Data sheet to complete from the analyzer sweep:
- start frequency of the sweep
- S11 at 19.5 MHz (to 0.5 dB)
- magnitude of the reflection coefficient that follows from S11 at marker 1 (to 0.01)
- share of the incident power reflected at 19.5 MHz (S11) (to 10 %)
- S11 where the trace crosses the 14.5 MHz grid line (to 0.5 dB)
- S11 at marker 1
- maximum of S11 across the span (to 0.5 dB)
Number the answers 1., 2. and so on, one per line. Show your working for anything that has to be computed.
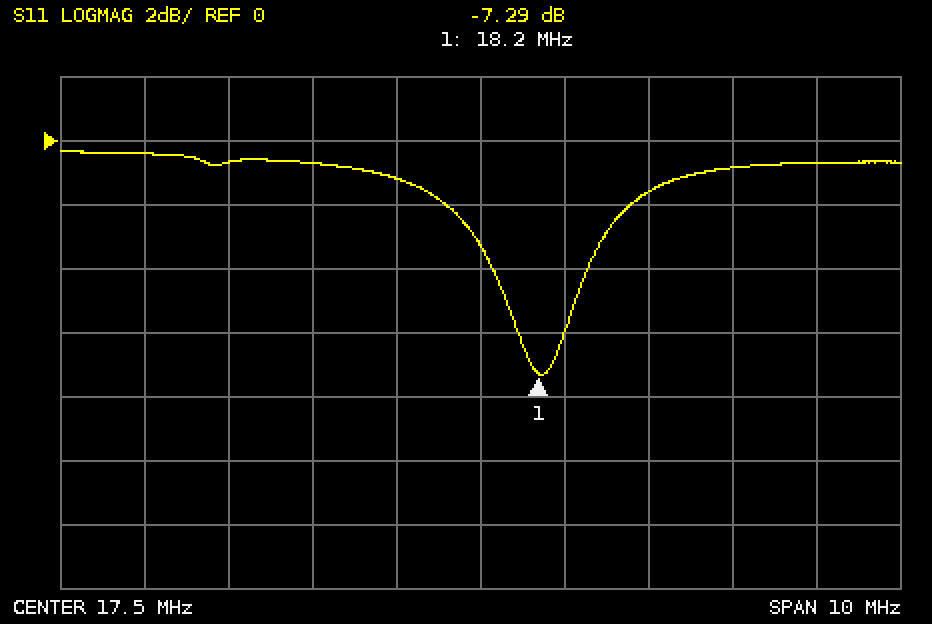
1. 12.5 MHz
2. -1.5 dB
3. 10^(-7.29/20) ≈ 0.43
4. 10^(-1.5/10) ≈ 70.8 %, so 70 % to the nearest 10 %
5. -0.5 dB
6. -7.29 dB
7. -0.5 dB
